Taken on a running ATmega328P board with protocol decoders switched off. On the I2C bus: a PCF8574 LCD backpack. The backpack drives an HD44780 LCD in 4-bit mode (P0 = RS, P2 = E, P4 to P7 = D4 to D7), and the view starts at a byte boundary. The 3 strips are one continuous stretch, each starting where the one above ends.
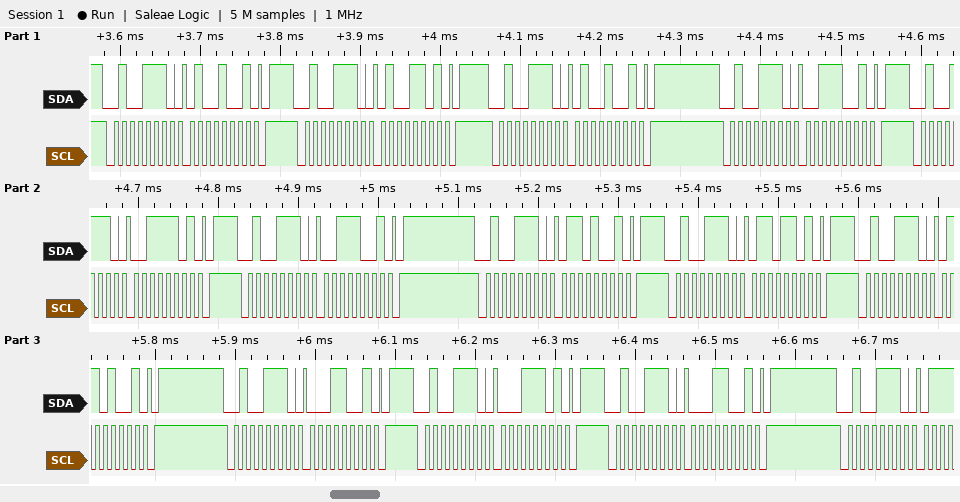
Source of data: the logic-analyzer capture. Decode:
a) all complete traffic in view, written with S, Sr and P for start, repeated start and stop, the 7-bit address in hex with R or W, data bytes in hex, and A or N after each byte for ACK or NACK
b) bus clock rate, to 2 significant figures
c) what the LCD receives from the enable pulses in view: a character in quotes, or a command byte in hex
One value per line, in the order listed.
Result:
S 27W A 49 A P S 27W A 4D A P S 27W A 49 A P S 27W A 39 A P S 27W A 3D A P S 27W A 39 A P S 27W A 69 A P S 27W A 6D A P S 27W A 69 A P S 27W A 19 A P S 27W A 1D A P S 27W A 19 A P S 27W A
100 kHz
'C' 'a'
